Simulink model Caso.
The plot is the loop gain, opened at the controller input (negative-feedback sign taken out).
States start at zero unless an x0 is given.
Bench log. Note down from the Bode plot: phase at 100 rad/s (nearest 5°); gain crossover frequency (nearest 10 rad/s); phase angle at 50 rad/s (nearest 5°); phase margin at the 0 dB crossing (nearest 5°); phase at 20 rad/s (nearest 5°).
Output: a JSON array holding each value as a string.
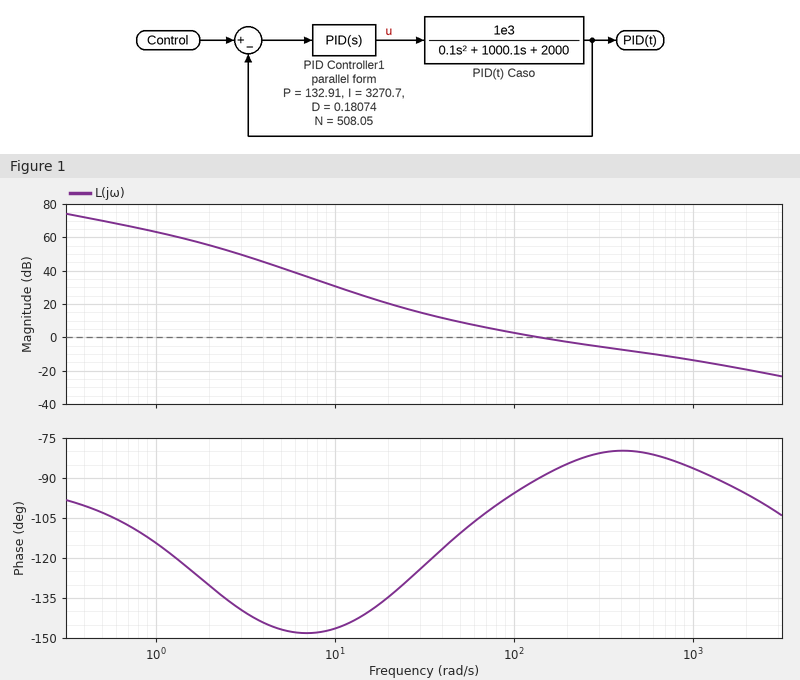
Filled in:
["-95°", "140 rad/s", "-110°", "90°", "-135°"]
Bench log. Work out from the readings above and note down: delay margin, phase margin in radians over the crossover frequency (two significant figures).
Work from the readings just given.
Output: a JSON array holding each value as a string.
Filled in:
["0.011 s"]
